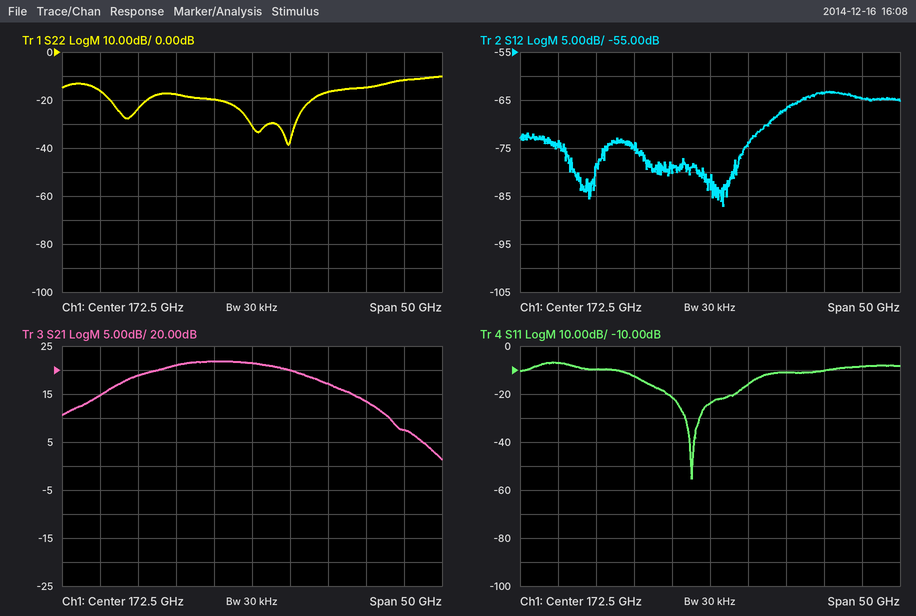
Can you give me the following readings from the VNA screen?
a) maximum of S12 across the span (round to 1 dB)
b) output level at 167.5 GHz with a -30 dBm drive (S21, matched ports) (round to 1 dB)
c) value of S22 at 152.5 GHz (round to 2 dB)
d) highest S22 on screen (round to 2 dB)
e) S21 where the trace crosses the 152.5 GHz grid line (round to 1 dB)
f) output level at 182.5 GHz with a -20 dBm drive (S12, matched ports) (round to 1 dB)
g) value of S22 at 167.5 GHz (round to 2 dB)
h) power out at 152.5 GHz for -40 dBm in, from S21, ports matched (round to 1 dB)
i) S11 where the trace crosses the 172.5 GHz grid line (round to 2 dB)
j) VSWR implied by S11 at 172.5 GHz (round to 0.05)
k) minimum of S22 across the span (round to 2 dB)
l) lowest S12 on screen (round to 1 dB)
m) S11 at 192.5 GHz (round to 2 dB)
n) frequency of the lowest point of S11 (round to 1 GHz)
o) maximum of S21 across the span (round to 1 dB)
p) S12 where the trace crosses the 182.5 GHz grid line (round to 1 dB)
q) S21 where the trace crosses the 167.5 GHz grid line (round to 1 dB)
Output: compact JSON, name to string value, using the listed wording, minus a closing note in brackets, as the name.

{"maximum of S12 across the span": "-63 dB", "output level at 167.5 GHz with a -30 dBm drive (S21, matched ports)": "-8 dBm", "value of S22 at 152.5 GHz": "-16 dB", "highest S22 on screen": "-10 dB", "S21 where the trace crosses the 152.5 GHz grid line": "15 dB", "output level at 182.5 GHz with a -20 dBm drive (S12, matched ports)": "-87 dBm", "value of S22 at 167.5 GHz": "-20 dB", "power out at 152.5 GHz for -40 dBm in, from S21, ports matched": "-25 dBm", "S11 where the trace crosses the 172.5 GHz grid line": "-24 dB", "VSWR implied by S11 at 172.5 GHz": "1.15", "minimum of S22 across the span": "-38 dB", "lowest S12 on screen": "-87 dB", "S11 at 192.5 GHz": "-8 dB", "frequency of the lowest point of S11": "170 GHz", "maximum of S21 across the span": "22 dB", "S12 where the trace crosses the 182.5 GHz grid line": "-67 dB", "S21 where the trace crosses the 167.5 GHz grid line": "22 dB"}
